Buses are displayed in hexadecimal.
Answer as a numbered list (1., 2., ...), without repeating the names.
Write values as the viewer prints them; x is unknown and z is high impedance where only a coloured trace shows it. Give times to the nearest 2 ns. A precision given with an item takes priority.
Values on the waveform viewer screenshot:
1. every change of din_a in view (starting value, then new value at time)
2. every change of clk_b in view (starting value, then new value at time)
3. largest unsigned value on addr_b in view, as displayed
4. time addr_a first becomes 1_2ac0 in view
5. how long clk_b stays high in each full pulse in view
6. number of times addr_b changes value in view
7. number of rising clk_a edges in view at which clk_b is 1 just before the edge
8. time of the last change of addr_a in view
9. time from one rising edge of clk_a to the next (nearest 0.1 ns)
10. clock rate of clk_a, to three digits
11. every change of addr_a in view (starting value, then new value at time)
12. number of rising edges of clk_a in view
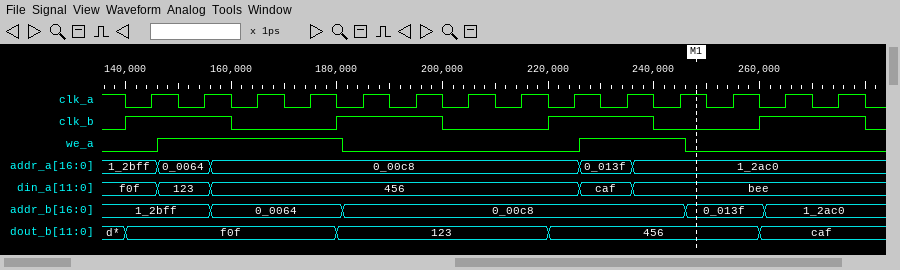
1. f0f, 123 at 146 ns, 456 at 156 ns, caf at 226 ns, bee at 236 ns
2. 0, 1 at 140 ns, 0 at 160 ns, 1 at 180 ns, 0 at 200 ns, 1 at 220 ns, 0 at 240 ns, 1 at 260 ns, 0 at 280 ns
3. 1_2bff
4. 236 ns
5. 20 ns, 20 ns, 20 ns, 20 ns
6. 4
7. 8
8. 236 ns
9. 10 ns
10. 100 MHz
11. 1_2bff, 0_0064 at 146 ns, 0_00c8 at 156 ns, 0_013f at 226 ns, 1_2ac0 at 236 ns
12. 14
